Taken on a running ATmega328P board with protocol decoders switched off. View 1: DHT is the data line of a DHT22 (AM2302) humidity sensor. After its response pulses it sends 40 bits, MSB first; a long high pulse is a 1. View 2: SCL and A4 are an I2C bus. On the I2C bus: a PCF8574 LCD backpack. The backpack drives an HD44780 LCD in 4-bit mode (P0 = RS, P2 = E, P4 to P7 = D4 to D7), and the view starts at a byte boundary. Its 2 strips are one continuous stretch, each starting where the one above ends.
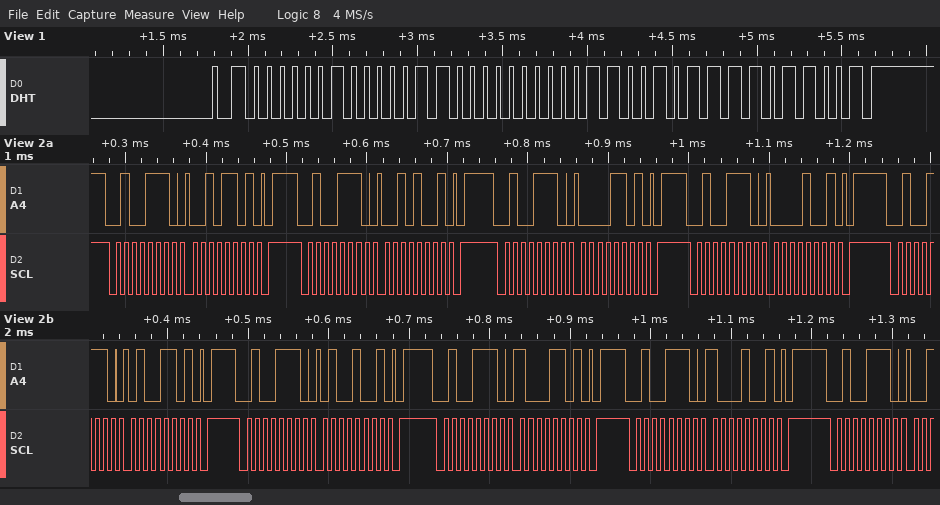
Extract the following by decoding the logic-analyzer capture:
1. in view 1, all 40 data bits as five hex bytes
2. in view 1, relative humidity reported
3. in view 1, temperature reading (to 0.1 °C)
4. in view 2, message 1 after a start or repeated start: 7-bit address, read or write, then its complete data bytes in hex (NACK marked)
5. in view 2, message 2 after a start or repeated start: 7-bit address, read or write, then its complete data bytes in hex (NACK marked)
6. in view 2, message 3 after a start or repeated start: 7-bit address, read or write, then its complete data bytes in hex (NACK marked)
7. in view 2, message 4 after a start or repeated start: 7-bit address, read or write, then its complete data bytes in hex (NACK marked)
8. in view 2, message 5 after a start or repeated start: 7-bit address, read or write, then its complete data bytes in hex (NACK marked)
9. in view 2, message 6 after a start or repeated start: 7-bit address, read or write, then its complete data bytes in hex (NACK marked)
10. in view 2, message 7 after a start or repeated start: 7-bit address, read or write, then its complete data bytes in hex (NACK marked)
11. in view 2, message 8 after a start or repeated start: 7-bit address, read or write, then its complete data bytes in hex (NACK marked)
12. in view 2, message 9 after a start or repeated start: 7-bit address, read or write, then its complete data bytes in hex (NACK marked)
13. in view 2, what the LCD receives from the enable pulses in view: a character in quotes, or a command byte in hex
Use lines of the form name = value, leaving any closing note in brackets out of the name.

in view 1, all 40 data bits as five hex bytes = 02 0C 00 CB D9
in view 1, relative humidity reported = 52.4 %
in view 1, temperature reading = 20.3 °C
in view 2, message 1 after a start or repeated start: 7-bit address, read or write, then its complete data bytes in hex = 0x27 write: 2D
in view 2, message 2 after a start or repeated start: 7-bit address, read or write, then its complete data bytes in hex = 0x27 write: 29
in view 2, message 3 after a start or repeated start: 7-bit address, read or write, then its complete data bytes in hex = 0x27 write: 0D
in view 2, message 4 after a start or repeated start: 7-bit address, read or write, then its complete data bytes in hex = 0x27 write: 09
in view 2, message 5 after a start or repeated start: 7-bit address, read or write, then its complete data bytes in hex = 0x27 write: 4D
in view 2, message 6 after a start or repeated start: 7-bit address, read or write, then its complete data bytes in hex = 0x27 write: 49
in view 2, message 7 after a start or repeated start: 7-bit address, read or write, then its complete data bytes in hex = 0x27 write: 8D
in view 2, message 8 after a start or repeated start: 7-bit address, read or write, then its complete data bytes in hex = 0x27 write: 89
in view 2, message 9 after a start or repeated start: 7-bit address, read or write, then its complete data bytes in hex = 0x27 write
in view 2, what the LCD receives from the enable pulses in view: a character in quotes, or a command byte in hex = ' ' 'H'
